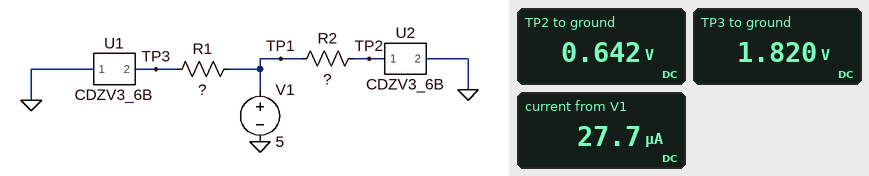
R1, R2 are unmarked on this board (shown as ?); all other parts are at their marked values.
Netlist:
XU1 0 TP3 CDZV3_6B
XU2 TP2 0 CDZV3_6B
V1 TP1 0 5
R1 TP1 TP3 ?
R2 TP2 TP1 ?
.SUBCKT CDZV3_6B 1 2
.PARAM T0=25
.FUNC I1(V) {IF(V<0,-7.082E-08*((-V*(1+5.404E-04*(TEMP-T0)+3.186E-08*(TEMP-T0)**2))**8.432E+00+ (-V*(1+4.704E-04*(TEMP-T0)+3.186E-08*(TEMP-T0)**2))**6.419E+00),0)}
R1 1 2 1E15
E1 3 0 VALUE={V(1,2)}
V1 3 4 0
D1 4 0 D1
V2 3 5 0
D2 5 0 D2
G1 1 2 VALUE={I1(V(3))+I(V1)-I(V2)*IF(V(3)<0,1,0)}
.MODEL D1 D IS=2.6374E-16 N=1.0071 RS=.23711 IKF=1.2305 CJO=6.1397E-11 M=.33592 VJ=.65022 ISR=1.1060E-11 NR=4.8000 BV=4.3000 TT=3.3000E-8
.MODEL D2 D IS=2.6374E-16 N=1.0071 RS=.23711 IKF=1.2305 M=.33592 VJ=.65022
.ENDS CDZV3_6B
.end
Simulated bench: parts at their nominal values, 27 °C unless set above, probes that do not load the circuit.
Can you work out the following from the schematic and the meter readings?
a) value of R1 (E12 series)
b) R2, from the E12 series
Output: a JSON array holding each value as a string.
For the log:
["220 kΩ", "330 kΩ"]
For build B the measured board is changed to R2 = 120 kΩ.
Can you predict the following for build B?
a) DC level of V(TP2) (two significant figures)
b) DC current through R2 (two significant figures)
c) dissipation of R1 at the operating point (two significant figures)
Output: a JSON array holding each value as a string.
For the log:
["670 mV", "36 µA", "46 µW"]
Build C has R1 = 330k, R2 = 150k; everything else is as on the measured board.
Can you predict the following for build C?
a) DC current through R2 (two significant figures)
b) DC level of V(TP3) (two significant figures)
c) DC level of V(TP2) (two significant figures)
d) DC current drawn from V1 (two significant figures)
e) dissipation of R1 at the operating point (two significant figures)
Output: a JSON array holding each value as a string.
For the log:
["29 µA", "1.7 V", "660 mV", "39 µA", "32 µW"]
